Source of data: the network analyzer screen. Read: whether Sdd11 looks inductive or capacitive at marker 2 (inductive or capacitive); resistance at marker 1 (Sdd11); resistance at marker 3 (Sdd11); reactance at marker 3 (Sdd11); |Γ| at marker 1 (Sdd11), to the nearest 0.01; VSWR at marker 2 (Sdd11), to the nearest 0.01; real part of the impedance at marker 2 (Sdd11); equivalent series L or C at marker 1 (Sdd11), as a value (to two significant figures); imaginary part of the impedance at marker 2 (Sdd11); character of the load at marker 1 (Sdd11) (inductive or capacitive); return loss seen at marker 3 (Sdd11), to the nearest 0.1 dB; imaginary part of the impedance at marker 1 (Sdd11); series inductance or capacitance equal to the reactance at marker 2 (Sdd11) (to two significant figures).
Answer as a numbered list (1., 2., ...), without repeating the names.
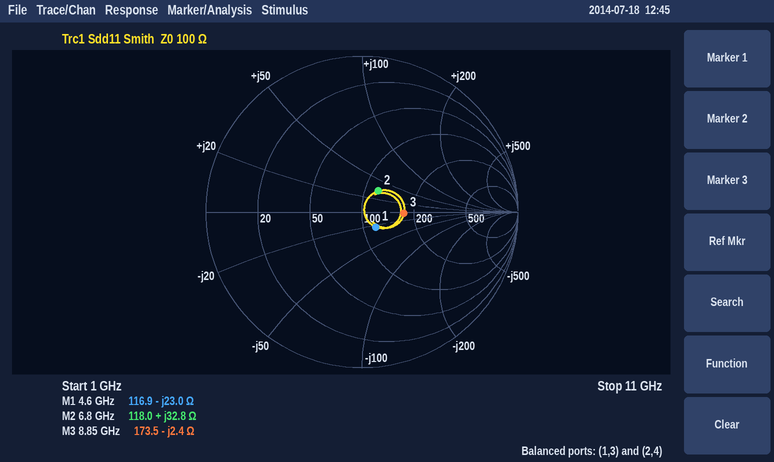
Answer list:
1. inductive
2. 116.9 Ω
3. 173.5 Ω
4. -2.4 Ω
5. 0.13
6. 1.41
7. 118.0 Ω
8. 1.5 pF
9. +32.8 Ω
10. capacitive
11. 11.4 dB
12. -23.0 Ω
13. 770 pH
